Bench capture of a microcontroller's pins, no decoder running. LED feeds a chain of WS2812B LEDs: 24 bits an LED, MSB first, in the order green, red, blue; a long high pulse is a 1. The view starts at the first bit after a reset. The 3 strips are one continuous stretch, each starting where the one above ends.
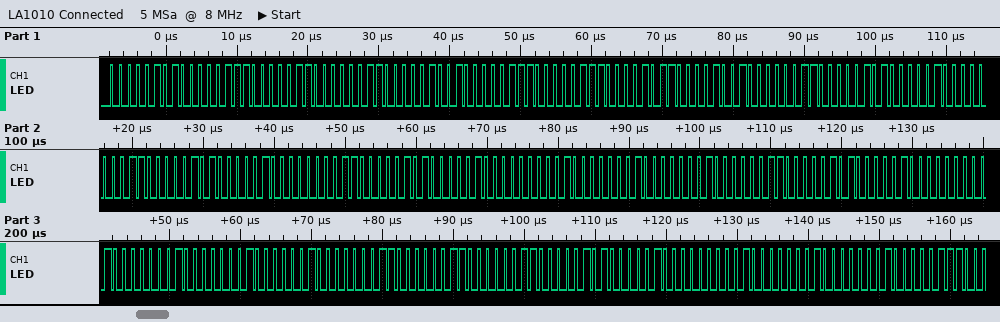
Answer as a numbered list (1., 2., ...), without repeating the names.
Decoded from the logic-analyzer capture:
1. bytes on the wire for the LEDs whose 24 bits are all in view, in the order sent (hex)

1. 05 07 06 06 09 07 07 0B 09 03 05 04 03 05 04 03 05 04 01 01 01 03 05 04 01 01 01 02 03 03 03 05 04 01 01 01
